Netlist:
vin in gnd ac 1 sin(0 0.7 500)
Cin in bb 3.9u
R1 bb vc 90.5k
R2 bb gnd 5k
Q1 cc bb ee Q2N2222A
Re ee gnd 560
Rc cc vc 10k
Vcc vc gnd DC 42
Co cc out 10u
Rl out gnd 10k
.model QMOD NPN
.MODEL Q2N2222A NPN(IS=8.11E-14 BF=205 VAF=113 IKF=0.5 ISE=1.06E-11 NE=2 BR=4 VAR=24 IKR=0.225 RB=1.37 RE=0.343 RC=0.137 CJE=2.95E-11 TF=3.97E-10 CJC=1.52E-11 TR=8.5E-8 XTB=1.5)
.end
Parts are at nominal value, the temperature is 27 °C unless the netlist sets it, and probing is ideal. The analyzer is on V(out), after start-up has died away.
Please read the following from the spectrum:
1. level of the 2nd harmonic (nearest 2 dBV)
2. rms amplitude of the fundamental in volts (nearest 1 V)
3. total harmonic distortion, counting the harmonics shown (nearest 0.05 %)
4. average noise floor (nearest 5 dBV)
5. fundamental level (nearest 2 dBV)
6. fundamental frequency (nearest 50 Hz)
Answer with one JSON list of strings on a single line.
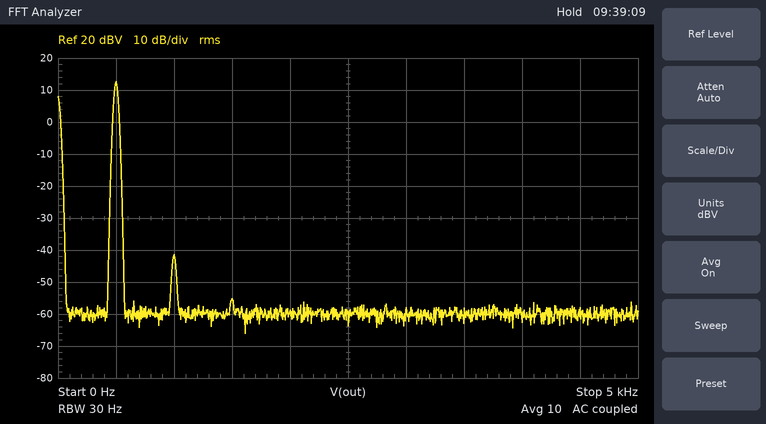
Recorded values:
["-42 dBV", "4 V", "0.20 %", "-60 dBV", "12 dBV", "500 Hz"]
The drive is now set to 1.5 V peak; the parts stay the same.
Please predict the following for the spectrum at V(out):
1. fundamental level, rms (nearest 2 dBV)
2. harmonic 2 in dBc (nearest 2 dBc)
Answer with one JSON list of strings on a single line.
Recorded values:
["20 dBV", "-46 dBc"]
